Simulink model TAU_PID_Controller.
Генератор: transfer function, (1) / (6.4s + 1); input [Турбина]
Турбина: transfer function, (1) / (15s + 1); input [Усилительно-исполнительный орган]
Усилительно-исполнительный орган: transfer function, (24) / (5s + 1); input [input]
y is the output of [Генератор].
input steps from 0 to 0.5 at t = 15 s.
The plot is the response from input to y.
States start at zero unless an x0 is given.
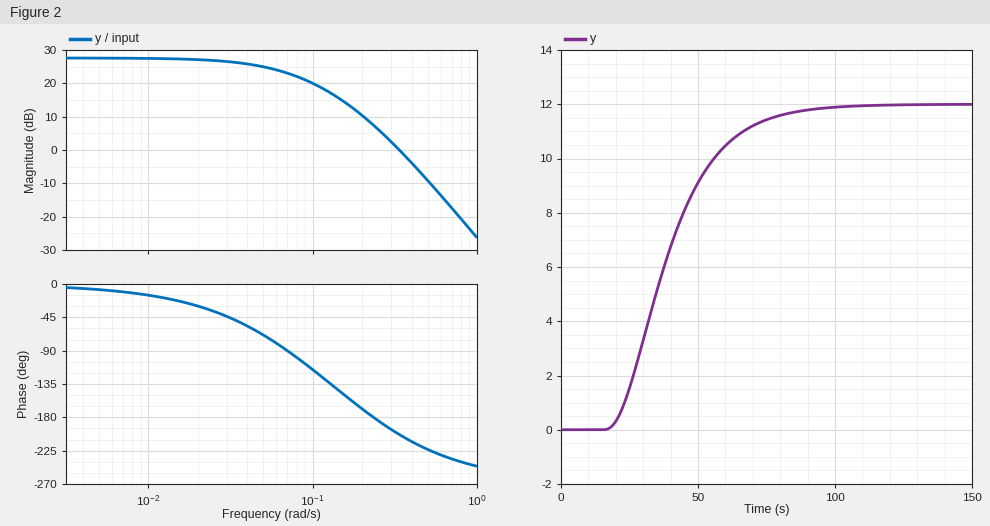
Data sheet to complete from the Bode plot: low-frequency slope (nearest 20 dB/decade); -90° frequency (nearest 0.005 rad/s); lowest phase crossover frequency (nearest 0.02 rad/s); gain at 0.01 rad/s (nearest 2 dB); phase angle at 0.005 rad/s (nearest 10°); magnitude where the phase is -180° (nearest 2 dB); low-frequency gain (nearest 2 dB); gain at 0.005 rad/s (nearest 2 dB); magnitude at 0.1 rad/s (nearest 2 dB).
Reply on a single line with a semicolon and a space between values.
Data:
0 dB/decade; 0.070 rad/s; 0.24 rad/s; 28 dB; -10°; 8 dB; 28 dB; 28 dB; 20 dB
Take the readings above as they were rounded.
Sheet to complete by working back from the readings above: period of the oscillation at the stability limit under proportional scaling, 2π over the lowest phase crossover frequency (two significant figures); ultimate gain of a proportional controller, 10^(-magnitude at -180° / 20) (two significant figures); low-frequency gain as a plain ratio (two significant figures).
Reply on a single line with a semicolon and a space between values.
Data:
26 s; 0.40; 25
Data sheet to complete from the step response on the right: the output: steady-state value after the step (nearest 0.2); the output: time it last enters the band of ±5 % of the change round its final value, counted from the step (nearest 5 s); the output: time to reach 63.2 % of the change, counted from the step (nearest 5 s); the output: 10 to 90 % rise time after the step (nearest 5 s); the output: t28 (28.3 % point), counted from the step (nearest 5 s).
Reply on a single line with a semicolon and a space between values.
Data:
12.0; 60 s; 30 s; 40 s; 15 s
